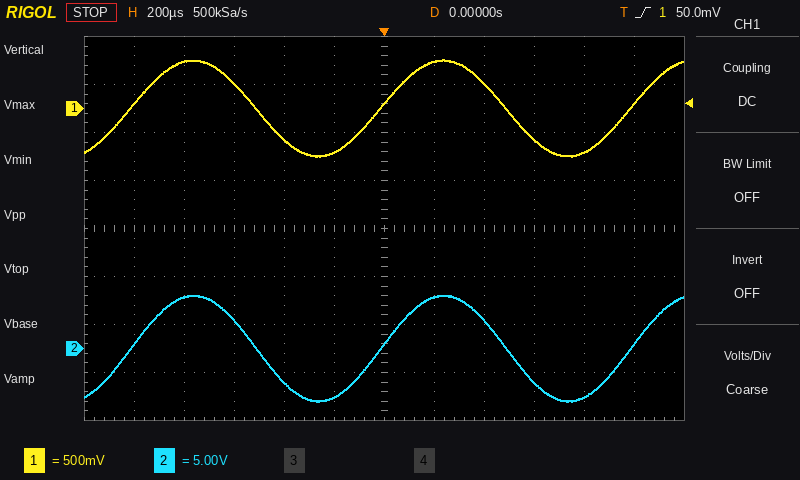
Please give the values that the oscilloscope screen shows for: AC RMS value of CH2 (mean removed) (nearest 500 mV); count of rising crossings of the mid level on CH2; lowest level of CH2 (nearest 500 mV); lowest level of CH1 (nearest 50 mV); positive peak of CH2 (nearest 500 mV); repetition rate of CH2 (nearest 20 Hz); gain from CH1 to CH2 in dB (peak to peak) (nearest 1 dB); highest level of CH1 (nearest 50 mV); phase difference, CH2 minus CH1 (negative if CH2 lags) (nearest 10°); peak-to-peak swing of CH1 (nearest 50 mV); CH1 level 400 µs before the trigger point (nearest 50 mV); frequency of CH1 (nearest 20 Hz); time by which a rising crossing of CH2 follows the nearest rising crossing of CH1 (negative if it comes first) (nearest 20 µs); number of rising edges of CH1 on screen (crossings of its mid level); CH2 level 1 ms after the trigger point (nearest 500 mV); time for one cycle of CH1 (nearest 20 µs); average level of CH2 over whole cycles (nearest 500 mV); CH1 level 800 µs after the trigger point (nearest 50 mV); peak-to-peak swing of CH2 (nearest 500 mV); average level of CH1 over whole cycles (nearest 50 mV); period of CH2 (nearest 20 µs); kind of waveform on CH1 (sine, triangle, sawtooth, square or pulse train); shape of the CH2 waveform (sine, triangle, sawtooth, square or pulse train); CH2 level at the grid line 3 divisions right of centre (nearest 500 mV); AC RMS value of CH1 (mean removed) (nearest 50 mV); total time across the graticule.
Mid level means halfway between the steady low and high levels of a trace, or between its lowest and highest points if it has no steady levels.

4.0 V
3
-5.5 V
-500 mV
5.5 V
1.00 kHz
21 dB
500 mV
0°
1.00 V
-300 mV
1.00 kHz
0 µs
3
500 mV
1.00 ms
0.0 V
-450 mV
11.0 V
0 mV
1.00 ms
sine
sine
-3.5 V
350 mV
2.4 ms
